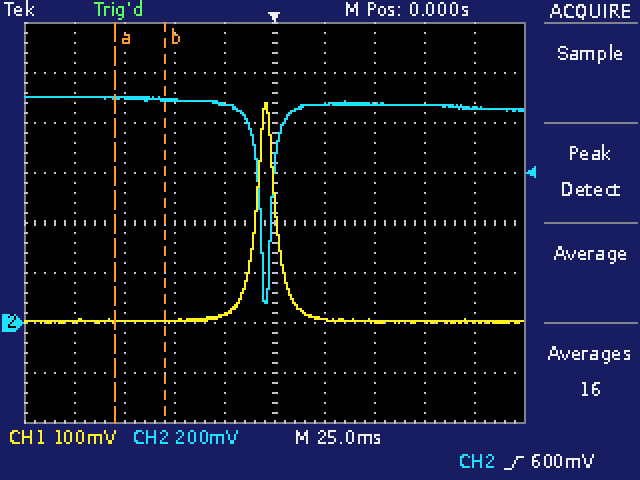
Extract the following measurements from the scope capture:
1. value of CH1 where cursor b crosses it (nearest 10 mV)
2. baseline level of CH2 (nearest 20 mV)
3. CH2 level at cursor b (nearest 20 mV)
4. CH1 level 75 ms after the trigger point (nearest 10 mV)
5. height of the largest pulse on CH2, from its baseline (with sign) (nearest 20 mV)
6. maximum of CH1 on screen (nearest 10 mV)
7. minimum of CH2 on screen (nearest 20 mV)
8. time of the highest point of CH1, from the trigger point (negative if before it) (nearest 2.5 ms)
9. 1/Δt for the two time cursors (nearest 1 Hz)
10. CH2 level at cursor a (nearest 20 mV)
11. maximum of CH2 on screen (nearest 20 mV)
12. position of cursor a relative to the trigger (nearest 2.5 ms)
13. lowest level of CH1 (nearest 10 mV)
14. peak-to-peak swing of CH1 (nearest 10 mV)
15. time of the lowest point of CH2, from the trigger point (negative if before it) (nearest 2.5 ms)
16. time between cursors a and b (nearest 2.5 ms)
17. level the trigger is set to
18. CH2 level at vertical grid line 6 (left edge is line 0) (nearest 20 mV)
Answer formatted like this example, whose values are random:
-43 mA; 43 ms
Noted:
0 mV; 880 mV; 900 mV; 0 mV; -800 mV; 440 mV; 80 mV; -5.0 ms; 40 Hz; 900 mV; 900 mV; -80.0 ms; 0 mV; 440 mV; -5.0 ms; 25.0 ms; 600 mV; 880 mV
